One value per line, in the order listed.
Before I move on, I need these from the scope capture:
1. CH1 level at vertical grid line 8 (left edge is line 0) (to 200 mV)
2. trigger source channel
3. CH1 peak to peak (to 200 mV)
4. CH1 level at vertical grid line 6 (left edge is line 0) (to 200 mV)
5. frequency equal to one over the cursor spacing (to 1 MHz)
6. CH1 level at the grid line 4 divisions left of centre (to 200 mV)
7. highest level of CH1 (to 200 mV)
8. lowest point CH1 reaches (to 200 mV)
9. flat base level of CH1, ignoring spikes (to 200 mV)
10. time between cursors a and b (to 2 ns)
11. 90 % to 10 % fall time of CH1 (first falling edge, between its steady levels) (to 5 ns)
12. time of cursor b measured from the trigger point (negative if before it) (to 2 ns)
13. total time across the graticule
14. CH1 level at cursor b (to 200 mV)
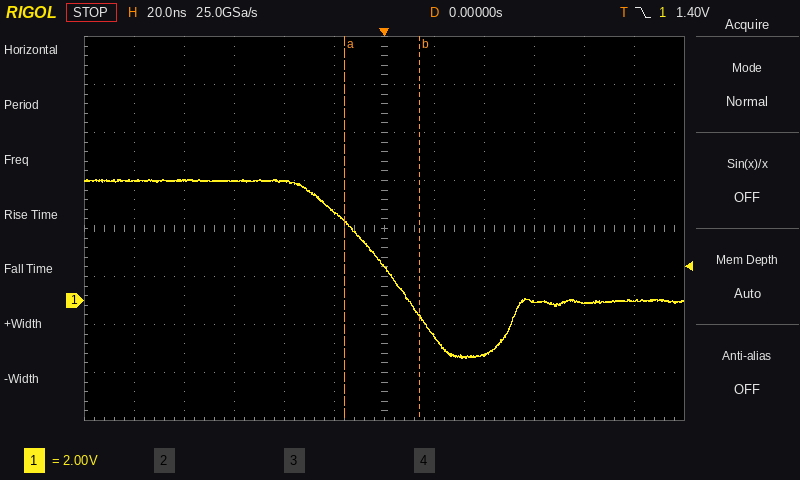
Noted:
-2.2 V
CH1
7.4 V
1.4 V
33 MHz
5.0 V
5.0 V
-2.4 V
0.0 V
30 ns
35 ns
+14 ns
240 ns
-600 mV
